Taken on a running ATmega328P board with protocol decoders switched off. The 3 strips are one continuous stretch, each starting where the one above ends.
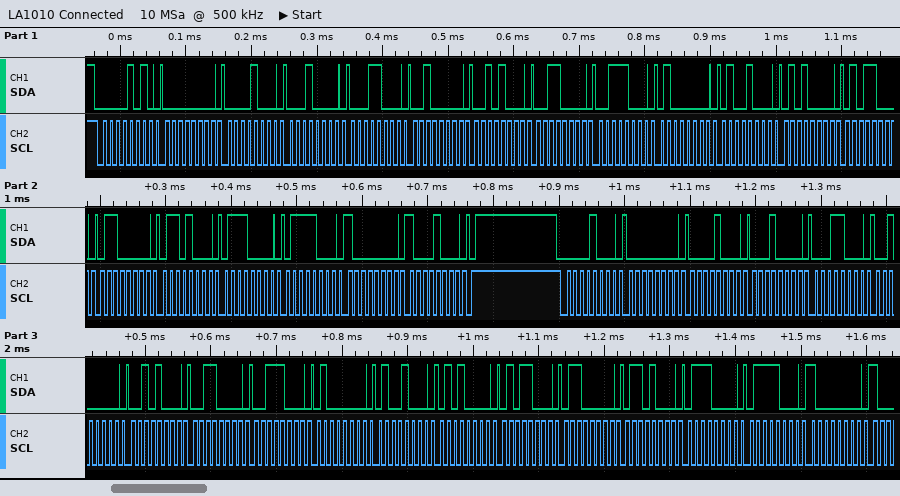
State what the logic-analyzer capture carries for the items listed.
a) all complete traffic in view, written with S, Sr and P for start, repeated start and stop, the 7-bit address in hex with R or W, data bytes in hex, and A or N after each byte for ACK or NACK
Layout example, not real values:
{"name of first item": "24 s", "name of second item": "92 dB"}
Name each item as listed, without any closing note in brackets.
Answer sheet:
{"all complete traffic in view, written with S, Sr and P for start, repeated start and stop, the 7-bit address in hex with R or W, data bytes in hex, and A or N after each byte for ACK or NACK": "S 05W A 00 A 08 A 10 A 18 A 20 A 28 A 30 A 38 A 40 A 48 A 50 A 58 A 60 A 68 A 70 A 78 A 80 A 88 A P S 04W A 00 A 08 A 10 A 18 A 20 A 28 A 30 A 38 A 40 A 48 A 50 A 58 A 60 A 68 A 70 A 78 A 80 A"}
